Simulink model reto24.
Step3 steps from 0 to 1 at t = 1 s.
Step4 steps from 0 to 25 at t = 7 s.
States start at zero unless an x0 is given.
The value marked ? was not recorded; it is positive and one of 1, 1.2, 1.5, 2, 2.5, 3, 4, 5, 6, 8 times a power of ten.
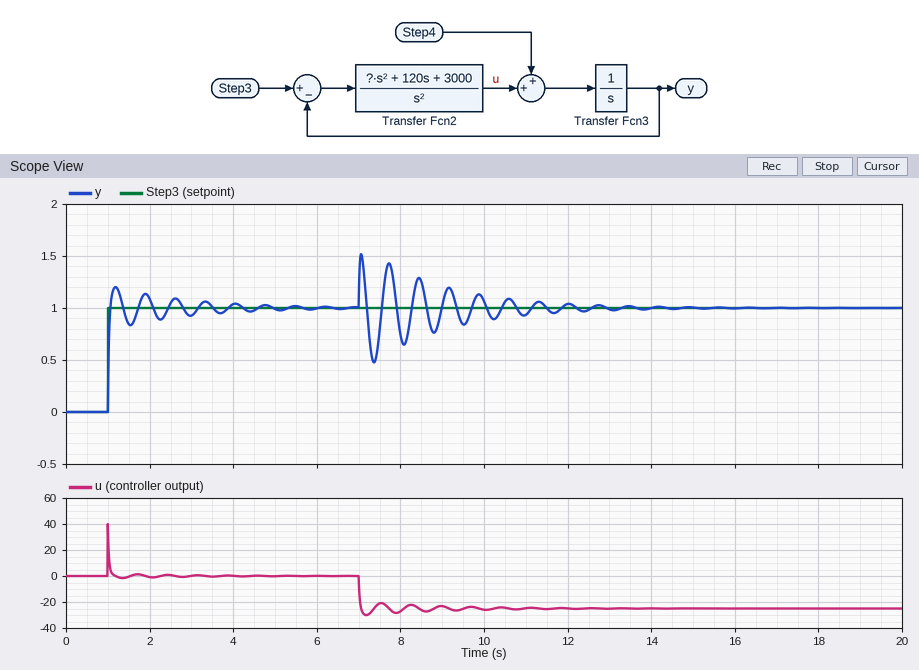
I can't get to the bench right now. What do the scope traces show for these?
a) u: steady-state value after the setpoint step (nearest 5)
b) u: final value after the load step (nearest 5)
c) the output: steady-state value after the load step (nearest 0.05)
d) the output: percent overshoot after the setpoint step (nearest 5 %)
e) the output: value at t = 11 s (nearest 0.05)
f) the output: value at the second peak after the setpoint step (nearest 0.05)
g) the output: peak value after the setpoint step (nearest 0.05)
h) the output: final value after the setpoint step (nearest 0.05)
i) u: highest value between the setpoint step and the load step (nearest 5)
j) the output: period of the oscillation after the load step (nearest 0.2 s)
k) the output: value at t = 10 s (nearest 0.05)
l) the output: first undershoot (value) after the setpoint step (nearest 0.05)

0
-25
1.00
20 %
0.95
1.15
1.20
1.00
40
0.8 s
1.05
0.85
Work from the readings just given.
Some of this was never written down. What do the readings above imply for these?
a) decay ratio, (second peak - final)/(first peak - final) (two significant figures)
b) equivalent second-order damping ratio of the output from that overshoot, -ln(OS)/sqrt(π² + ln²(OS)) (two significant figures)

0.75
0.46
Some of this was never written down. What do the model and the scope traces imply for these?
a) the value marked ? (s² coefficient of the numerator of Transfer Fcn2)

40
